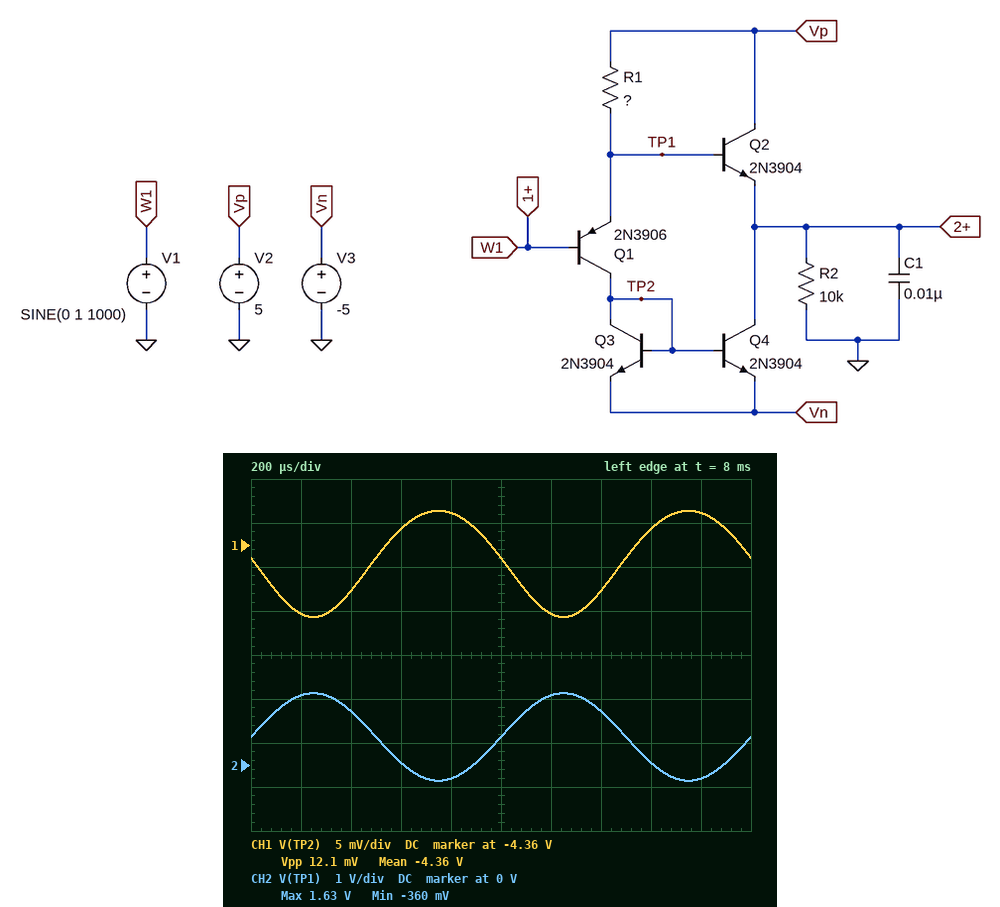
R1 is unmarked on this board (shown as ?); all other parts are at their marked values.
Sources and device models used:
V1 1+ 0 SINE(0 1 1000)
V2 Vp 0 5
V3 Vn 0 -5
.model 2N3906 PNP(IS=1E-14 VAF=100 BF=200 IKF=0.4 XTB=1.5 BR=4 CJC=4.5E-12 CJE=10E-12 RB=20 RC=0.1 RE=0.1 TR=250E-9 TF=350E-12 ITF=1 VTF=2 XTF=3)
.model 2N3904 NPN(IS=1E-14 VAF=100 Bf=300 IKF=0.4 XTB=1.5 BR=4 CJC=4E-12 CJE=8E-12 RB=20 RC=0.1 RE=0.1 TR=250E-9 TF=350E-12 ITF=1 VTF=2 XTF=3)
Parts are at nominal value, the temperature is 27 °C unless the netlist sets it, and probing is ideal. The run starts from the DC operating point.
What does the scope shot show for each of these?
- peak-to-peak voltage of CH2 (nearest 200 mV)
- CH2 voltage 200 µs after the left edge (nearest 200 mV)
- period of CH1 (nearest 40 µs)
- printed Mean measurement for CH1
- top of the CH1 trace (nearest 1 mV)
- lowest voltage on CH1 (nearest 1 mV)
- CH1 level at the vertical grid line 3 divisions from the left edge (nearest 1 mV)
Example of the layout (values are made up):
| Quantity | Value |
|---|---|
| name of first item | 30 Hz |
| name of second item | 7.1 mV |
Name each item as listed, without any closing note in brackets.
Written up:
| Quantity | Value |
|---|---|
| peak-to-peak voltage of CH2 | 2.0 V |
| CH2 voltage 200 µs after the left edge | 1.6 V |
| period of CH1 | 1.00 ms |
| printed Mean measurement for CH1 | -4.36 V |
| top of the CH1 trace | -4.356 V |
| lowest voltage on CH1 | -4.368 V |
| CH1 level at the vertical grid line 3 divisions from the left edge | -4.358 V |
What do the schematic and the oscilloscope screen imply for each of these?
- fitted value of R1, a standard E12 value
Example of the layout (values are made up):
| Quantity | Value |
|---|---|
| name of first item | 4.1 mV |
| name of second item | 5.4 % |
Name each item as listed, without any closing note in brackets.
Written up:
| Quantity | Value |
|---|---|
| fitted value of R1, a standard E12 value | 8.2 kΩ |
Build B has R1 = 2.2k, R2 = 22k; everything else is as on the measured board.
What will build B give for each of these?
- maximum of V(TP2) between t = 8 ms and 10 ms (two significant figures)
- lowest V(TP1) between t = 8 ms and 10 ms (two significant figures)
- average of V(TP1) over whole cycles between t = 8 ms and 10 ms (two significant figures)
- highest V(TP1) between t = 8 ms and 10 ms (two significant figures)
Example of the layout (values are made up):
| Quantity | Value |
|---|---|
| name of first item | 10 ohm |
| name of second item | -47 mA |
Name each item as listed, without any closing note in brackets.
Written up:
| Quantity | Value |
|---|---|
| maximum of V(TP2) between t = 8 ms and 10 ms | -4.3 V |
| lowest V(TP1) between t = 8 ms and 10 ms | -320 mV |
| average of V(TP1) over whole cycles between t = 8 ms and 10 ms | 670 mV |
| highest V(TP1) between t = 8 ms and 10 ms | 1.7 V |
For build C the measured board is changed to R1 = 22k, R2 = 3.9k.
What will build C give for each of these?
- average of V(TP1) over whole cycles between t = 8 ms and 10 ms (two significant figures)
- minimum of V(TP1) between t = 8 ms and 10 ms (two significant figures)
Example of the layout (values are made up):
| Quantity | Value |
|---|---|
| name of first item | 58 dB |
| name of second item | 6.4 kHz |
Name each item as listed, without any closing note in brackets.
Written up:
| Quantity | Value |
|---|---|
| average of V(TP1) over whole cycles between t = 8 ms and 10 ms | 610 mV |
| minimum of V(TP1) between t = 8 ms and 10 ms | -380 mV |
